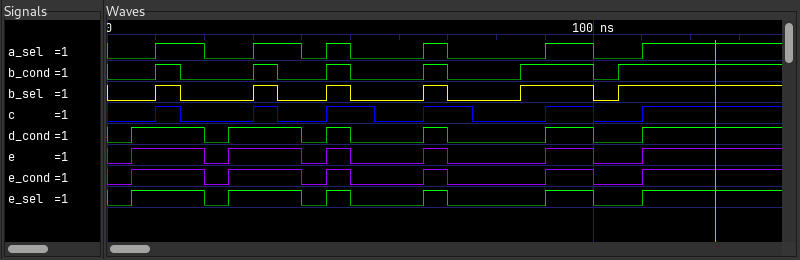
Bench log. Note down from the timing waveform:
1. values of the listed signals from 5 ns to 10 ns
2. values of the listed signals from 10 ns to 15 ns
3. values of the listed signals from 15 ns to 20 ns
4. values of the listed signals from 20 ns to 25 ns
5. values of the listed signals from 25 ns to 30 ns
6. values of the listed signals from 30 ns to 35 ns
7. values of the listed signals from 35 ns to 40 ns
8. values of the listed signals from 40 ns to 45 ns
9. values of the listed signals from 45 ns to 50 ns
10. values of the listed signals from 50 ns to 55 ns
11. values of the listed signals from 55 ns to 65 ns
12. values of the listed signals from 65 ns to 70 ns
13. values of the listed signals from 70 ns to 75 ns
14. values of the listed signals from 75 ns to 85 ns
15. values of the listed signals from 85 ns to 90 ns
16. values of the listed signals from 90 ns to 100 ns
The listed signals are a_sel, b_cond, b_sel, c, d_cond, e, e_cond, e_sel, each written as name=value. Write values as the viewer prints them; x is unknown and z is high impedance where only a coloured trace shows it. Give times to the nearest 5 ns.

a_sel=0, b_cond=0, b_sel=0, c=0, d_cond=1, e=1, e_cond=1, e_sel=1
a_sel=1, b_cond=1, b_sel=1, c=1, d_cond=1, e=1, e_cond=1, e_sel=1
a_sel=1, b_cond=0, b_sel=0, c=0, d_cond=1, e=1, e_cond=1, e_sel=1
a_sel=0, b_cond=0, b_sel=0, c=0, d_cond=0, e=0, e_cond=0, e_sel=0
a_sel=0, b_cond=0, b_sel=0, c=0, d_cond=1, e=1, e_cond=1, e_sel=1
a_sel=1, b_cond=1, b_sel=1, c=1, d_cond=1, e=1, e_cond=1, e_sel=1
a_sel=1, b_cond=0, b_sel=0, c=0, d_cond=1, e=1, e_cond=1, e_sel=1
a_sel=0, b_cond=0, b_sel=0, c=0, d_cond=0, e=0, e_cond=0, e_sel=0
a_sel=1, b_cond=1, b_sel=1, c=1, d_cond=1, e=1, e_cond=1, e_sel=1
a_sel=0, b_cond=0, b_sel=0, c=1, d_cond=0, e=0, e_cond=0, e_sel=0
a_sel=0, b_cond=0, b_sel=0, c=0, d_cond=0, e=0, e_cond=0, e_sel=0
a_sel=1, b_cond=1, b_sel=1, c=1, d_cond=1, e=1, e_cond=1, e_sel=1
a_sel=0, b_cond=0, b_sel=0, c=1, d_cond=0, e=0, e_cond=0, e_sel=0
a_sel=0, b_cond=0, b_sel=0, c=0, d_cond=0, e=0, e_cond=0, e_sel=0
a_sel=0, b_cond=1, b_sel=1, c=0, d_cond=0, e=0, e_cond=0, e_sel=0
a_sel=1, b_cond=1, b_sel=1, c=1, d_cond=1, e=1, e_cond=1, e_sel=1
